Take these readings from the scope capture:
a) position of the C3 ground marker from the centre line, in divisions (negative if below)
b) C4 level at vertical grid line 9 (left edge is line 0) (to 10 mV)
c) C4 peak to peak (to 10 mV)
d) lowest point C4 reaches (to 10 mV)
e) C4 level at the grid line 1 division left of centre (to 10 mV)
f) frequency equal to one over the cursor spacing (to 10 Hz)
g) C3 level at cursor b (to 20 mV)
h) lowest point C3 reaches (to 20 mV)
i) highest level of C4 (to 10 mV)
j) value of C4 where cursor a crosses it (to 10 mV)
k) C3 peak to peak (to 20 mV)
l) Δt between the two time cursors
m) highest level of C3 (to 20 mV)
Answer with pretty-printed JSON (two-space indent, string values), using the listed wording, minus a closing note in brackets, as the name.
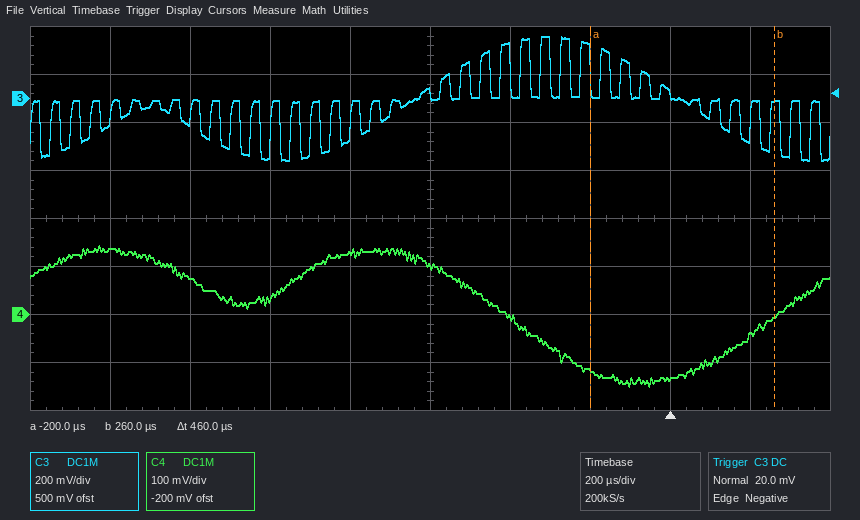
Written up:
{
  "position of the C3 ground marker from the centre line, in divisions": "+2.5 div",
  "C4 level at vertical grid line 9 (left edge is line 0)": "-50 mV",
  "C4 peak to peak": "290 mV",
  "lowest point C4 reaches": "-150 mV",
  "C4 level at the grid line 1 division left of centre": "130 mV",
  "frequency equal to one over the cursor spacing": "2.17 kHz",
  "C3 level at cursor b": "-20 mV",
  "lowest point C3 reaches": "-260 mV",
  "highest level of C4": "140 mV",
  "value of C4 where cursor a crosses it": "-120 mV",
  "C3 peak to peak": "520 mV",
  "Δt between the two time cursors": "460 µs",
  "highest level of C3": "260 mV"
}
